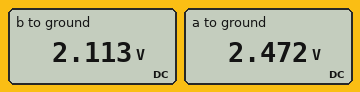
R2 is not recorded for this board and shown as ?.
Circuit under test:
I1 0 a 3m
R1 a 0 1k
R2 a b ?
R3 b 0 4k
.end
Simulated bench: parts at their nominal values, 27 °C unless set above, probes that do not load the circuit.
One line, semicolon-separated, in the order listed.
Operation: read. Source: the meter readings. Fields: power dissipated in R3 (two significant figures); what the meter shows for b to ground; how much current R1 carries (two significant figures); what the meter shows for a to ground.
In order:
1.1 mW; 2.113 V; 2.5 mA; 2.472 V
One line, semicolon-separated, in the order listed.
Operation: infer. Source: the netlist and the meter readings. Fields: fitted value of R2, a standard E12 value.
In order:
680 Ω
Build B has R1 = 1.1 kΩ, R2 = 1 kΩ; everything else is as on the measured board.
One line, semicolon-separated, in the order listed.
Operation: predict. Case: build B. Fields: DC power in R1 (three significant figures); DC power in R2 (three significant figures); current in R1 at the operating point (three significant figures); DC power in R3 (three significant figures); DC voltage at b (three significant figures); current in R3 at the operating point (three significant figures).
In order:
6.65 mW; 293 µW; 2.46 mA; 1.17 mW; 2.16 V; 541 µA
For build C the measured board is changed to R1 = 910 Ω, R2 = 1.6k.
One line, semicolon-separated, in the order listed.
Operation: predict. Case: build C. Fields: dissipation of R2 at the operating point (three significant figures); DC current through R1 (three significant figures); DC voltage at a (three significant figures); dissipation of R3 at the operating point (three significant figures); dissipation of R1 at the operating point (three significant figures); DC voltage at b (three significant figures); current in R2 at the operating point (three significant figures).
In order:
281 µW; 2.58 mA; 2.35 V; 703 µW; 6.06 mW; 1.68 V; 419 µA
